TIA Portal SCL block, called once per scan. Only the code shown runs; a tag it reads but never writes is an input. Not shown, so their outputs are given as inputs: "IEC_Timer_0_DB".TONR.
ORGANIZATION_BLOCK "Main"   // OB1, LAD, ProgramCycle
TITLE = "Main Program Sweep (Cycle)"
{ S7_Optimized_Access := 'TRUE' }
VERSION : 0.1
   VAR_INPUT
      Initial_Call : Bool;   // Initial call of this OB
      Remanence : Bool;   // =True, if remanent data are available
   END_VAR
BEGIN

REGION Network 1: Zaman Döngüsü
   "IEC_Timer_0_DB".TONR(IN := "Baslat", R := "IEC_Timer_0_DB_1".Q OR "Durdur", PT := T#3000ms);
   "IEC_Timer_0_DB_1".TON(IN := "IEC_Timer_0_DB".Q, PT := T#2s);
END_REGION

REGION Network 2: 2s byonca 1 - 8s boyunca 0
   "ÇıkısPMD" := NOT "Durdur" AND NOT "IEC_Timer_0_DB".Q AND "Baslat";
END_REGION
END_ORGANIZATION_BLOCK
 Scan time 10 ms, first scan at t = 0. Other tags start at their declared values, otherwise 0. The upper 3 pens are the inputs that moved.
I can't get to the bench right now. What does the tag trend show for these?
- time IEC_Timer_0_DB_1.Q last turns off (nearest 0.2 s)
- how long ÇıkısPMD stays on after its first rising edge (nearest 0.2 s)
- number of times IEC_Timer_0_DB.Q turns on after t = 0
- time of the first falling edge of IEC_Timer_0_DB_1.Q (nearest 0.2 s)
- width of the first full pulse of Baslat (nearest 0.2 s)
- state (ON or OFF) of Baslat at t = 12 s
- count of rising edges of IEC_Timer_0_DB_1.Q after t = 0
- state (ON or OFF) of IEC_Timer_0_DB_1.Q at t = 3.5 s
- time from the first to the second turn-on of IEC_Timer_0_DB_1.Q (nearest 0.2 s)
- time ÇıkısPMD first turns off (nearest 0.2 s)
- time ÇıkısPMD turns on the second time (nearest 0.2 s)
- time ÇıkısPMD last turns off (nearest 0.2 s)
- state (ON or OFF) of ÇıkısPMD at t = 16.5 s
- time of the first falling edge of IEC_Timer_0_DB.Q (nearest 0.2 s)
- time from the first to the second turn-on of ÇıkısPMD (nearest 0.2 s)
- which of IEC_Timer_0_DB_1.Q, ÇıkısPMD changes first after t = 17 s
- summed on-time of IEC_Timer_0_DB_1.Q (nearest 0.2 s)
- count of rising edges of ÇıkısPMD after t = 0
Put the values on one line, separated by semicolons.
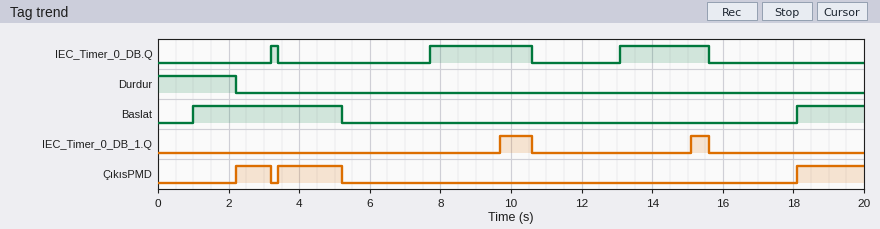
15.6 s; 1.0 s; 3; 10.6 s; 4.2 s; OFF; 2; OFF; 5.4 s; 3.2 s; 3.4 s; 5.2 s; OFF; 3.4 s; 1.2 s; ÇıkısPMD; 1.4 s; 3
